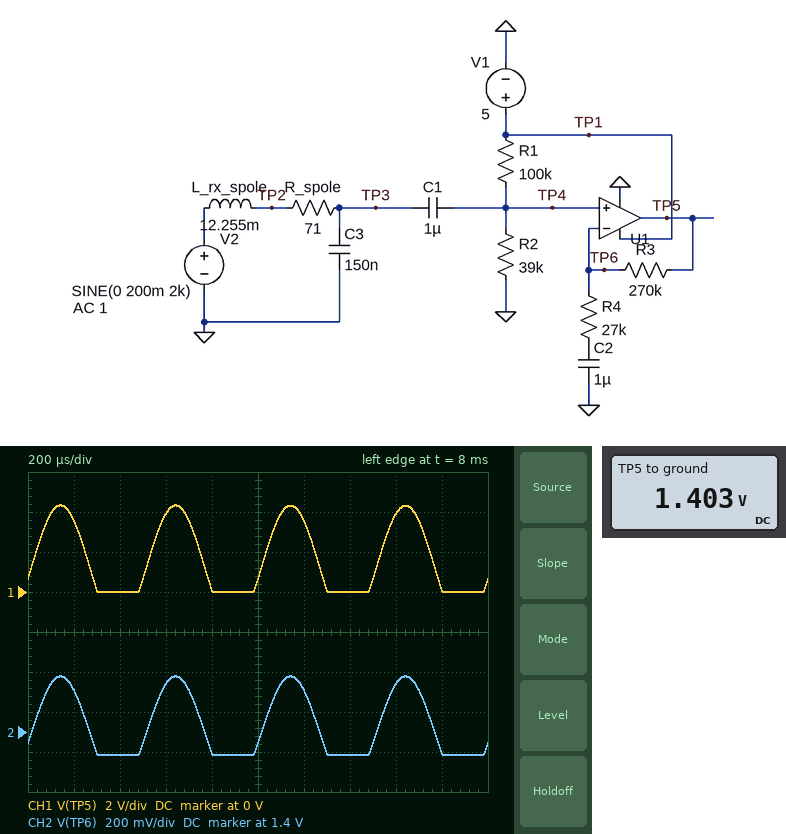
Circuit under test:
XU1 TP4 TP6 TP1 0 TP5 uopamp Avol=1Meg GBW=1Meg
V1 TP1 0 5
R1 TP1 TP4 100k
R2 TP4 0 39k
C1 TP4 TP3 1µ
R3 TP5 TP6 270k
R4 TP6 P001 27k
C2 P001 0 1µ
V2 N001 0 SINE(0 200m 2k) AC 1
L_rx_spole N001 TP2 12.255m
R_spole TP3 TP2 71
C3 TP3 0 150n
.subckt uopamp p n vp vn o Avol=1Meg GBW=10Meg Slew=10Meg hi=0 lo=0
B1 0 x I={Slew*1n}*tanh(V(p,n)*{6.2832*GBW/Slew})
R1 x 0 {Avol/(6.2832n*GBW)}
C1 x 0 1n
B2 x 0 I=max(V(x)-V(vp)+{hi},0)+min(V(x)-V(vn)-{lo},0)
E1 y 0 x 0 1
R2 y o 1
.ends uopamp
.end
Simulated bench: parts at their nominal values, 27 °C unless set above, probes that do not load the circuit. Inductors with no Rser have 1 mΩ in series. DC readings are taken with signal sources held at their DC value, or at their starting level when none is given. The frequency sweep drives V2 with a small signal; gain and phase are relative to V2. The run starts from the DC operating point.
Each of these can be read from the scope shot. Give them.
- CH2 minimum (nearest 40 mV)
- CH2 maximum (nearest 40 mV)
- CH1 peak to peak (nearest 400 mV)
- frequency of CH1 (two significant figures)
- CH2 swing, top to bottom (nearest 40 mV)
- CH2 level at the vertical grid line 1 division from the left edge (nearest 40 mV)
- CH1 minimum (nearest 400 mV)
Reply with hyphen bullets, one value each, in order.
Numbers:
- 1.28 V
- 1.68 V
- 4.4 V
- 2.0 kHz
- 400 mV
- 1.60 V
- 0 V
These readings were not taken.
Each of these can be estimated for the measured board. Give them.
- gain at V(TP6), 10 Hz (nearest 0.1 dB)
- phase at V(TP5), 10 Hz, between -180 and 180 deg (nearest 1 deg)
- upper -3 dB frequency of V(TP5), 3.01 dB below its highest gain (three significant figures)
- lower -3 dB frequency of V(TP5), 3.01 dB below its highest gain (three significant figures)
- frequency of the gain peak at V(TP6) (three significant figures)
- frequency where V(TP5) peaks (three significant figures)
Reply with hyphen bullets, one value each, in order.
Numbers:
- -1.2 dB
- 57 deg
- 4.11 kHz
- 3.13 kHz
- 3.65 kHz
- 3.65 kHz
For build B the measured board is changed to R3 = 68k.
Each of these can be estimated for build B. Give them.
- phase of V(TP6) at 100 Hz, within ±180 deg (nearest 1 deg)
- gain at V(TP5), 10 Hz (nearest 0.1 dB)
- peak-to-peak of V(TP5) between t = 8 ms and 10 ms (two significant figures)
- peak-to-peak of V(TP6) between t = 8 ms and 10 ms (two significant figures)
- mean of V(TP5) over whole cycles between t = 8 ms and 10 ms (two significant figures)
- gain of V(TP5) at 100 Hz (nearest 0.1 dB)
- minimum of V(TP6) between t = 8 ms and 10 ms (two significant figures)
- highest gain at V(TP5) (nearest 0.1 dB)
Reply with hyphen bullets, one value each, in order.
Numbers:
- 3 deg
- 8.5 dB
- 1.9 V
- 550 mV
- 1.4 V
- 10.9 dB
- 1.1 V
- 22.7 dB
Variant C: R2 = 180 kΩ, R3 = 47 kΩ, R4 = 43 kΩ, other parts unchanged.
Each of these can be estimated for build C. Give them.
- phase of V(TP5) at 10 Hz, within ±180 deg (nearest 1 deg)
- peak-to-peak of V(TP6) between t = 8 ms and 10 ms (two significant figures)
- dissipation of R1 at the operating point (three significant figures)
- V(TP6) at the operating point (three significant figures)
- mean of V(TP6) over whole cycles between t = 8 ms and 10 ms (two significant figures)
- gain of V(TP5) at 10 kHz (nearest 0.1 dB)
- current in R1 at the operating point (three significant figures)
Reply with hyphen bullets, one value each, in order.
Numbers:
- 24 deg
- 550 mV
- 31.9 µW
- 3.21 V
- 3.2 V
- -9.6 dB
- 17.9 µA
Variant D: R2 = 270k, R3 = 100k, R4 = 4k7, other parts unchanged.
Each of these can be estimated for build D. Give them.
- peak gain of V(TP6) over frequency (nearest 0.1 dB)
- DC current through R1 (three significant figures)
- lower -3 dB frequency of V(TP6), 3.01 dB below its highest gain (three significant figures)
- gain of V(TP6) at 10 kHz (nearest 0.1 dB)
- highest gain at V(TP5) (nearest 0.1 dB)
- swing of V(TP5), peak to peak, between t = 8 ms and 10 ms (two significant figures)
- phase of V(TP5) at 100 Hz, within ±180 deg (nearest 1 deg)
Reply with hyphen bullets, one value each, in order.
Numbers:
- 12.0 dB
- 13.5 µA
- 3.15 kHz
- -16.2 dB
- 39.0 dB
- 5.0 V
- 19 deg
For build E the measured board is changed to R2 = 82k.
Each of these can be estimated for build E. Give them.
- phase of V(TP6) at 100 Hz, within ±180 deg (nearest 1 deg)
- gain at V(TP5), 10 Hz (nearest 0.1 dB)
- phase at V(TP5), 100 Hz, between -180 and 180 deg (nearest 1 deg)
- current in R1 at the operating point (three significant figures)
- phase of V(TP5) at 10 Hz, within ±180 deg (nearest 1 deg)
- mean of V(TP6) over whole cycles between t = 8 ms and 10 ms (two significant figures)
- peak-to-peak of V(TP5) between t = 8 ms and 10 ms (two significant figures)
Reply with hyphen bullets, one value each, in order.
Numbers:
- 2 deg
- 19.0 dB
- 5 deg
- 27.5 µA
- 47 deg
- 2.3 V
- 5.0 V
